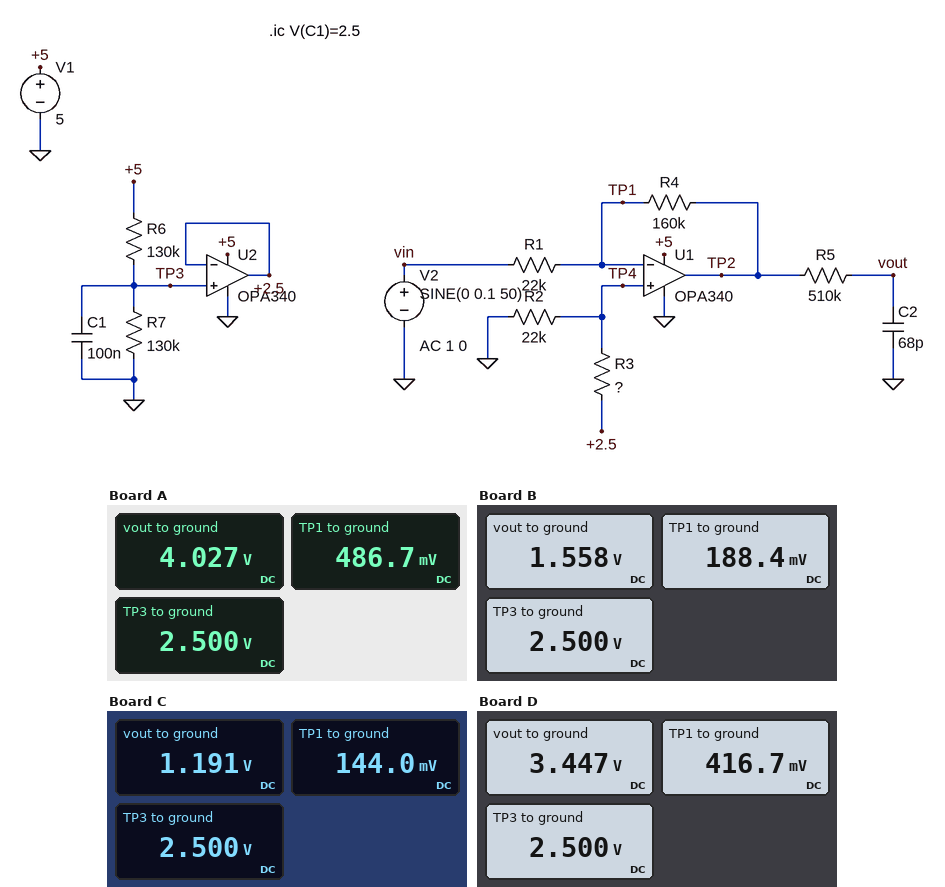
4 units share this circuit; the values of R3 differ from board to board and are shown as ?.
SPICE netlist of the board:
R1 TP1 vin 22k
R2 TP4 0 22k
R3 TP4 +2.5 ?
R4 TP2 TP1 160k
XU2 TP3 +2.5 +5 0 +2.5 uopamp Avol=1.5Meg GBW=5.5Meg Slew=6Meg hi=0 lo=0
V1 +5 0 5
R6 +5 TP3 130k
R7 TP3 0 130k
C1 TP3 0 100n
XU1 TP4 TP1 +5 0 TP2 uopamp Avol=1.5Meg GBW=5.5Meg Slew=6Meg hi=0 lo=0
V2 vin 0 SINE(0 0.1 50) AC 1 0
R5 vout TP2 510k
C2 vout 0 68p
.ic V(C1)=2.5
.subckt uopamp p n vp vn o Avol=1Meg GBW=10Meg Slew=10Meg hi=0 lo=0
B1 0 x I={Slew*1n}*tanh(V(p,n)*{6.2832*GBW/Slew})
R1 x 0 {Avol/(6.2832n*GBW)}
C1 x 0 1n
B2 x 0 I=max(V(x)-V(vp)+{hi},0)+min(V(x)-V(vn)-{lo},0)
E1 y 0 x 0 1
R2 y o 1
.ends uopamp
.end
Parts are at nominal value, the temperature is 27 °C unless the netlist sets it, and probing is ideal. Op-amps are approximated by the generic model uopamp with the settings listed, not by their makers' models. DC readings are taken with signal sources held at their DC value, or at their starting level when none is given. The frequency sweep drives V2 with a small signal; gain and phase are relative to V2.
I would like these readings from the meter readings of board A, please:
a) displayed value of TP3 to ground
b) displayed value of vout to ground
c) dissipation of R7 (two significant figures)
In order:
2.500 V
4.027 V
48 µW
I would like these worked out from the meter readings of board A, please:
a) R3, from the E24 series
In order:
91 kΩ
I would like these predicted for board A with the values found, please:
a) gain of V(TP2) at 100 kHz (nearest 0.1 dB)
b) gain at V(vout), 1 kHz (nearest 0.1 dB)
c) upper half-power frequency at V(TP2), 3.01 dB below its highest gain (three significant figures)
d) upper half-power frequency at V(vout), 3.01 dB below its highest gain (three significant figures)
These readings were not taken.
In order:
17.1 dB
17.0 dB
665 kHz
4.59 kHz
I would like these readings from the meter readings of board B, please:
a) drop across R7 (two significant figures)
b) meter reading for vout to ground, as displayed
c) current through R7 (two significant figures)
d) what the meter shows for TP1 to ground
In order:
2.5 V
1.558 V
19 µA
188.4 mV
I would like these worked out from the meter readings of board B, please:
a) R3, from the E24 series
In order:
270 kΩ
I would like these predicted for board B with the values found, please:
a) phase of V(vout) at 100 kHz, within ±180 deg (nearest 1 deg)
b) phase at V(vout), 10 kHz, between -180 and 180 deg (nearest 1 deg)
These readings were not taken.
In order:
84 deg
114 deg
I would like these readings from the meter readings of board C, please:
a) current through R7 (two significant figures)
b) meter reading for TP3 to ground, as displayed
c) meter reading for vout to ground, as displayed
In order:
19 µA
2.500 V
1.191 V
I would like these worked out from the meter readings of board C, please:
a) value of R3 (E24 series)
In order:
360 kΩ
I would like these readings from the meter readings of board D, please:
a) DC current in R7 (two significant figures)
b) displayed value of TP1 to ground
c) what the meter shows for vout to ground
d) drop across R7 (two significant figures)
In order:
19 µA
416.7 mV
3.447 V
2.5 V
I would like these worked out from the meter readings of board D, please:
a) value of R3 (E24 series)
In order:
110 kΩ
